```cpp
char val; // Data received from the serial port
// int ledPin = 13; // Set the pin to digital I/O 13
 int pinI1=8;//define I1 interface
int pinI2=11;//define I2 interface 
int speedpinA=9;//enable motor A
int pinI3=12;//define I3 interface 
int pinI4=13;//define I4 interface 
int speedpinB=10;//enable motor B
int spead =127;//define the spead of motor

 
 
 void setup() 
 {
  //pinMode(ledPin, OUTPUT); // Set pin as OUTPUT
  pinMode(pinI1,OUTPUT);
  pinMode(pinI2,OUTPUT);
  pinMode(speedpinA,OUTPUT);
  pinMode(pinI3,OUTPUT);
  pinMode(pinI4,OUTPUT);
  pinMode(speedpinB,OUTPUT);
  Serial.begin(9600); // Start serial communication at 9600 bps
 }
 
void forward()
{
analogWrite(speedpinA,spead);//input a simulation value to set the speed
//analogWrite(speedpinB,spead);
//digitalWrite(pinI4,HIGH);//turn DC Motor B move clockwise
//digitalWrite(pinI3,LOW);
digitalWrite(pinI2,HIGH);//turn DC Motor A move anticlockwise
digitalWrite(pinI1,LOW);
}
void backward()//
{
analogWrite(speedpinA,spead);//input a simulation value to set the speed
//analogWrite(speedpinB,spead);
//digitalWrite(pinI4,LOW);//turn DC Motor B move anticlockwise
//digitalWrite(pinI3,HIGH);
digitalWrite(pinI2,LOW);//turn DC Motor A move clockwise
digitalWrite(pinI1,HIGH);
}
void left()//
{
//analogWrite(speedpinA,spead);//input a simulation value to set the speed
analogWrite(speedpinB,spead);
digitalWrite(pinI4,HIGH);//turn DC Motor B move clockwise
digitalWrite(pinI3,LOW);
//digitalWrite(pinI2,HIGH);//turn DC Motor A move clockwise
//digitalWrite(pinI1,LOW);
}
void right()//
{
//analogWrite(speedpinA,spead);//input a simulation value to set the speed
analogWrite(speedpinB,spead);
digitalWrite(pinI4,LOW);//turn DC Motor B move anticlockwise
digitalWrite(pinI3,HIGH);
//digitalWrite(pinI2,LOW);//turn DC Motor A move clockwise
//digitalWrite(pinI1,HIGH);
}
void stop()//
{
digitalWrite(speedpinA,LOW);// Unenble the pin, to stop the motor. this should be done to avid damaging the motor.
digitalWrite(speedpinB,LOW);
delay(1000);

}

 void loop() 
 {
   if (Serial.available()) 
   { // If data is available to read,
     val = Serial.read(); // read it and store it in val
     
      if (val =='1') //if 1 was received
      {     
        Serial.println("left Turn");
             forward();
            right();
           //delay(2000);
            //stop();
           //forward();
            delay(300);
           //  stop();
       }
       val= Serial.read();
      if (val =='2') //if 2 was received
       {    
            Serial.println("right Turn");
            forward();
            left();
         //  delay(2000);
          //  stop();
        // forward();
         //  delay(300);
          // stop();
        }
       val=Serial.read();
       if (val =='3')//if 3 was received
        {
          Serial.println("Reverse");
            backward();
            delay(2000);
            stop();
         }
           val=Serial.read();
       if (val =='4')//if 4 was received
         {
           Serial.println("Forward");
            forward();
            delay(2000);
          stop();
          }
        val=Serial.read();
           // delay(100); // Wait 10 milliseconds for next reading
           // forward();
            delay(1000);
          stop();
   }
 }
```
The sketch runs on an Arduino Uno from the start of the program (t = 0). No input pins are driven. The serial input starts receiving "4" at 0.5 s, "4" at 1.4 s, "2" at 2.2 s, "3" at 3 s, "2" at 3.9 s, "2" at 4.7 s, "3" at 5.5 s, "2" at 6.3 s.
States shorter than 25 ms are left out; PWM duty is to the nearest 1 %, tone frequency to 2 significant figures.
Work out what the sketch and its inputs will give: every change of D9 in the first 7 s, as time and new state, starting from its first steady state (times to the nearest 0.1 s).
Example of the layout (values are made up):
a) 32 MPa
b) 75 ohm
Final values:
a) 0 s low; 2.5 s PWM 50 %; 3.5 s low; 4.5 s PWM 50 %; 5.5 s low
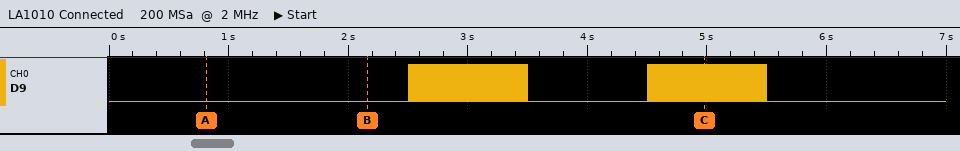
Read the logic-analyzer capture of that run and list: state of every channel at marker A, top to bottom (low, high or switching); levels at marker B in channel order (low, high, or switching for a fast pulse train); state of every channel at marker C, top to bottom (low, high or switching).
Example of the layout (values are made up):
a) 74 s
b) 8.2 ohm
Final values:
a) D9 low
b) D9 low
c) D9 switching
